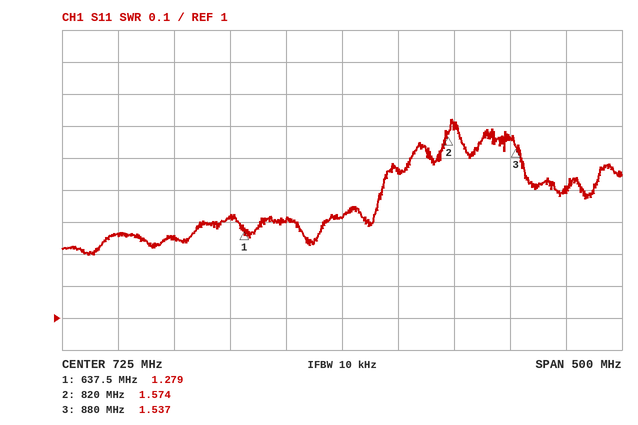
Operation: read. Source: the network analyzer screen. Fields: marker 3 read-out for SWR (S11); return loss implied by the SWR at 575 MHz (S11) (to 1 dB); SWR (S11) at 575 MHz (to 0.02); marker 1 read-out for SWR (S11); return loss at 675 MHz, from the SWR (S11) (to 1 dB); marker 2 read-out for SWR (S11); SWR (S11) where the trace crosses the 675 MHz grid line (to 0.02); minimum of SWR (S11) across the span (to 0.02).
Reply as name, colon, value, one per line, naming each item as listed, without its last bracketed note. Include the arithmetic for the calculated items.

marker 3 read-out for SWR: 1.537
return loss implied by the SWR at 575 MHz (S11): −20 log10((1.26 − 1)/(1.26 + 1)) ≈ 19 dB
SWR (S11) at 575 MHz: 1.26
marker 1 read-out for SWR: 1.279
return loss at 675 MHz, from the SWR (S11): −20 log10((1.3 − 1)/(1.3 + 1)) ≈ 18 dB
marker 2 read-out for SWR: 1.574
SWR (S11) where the trace crosses the 675 MHz grid line: 1.30
minimum of SWR (S11) across the span: 1.20
